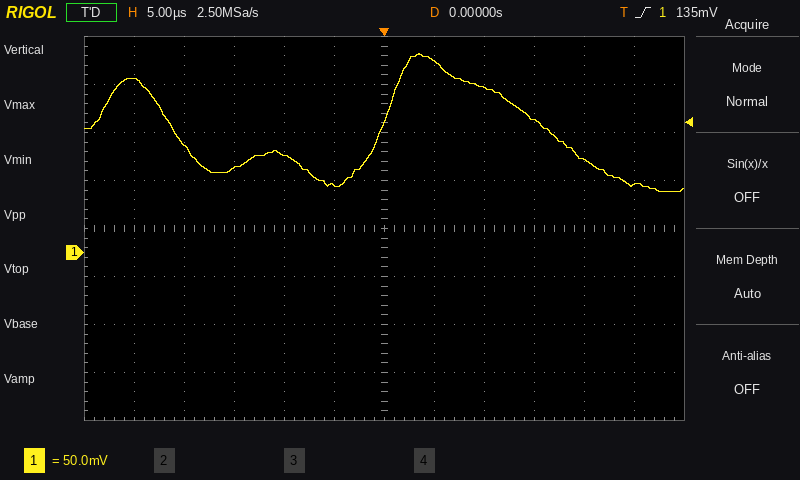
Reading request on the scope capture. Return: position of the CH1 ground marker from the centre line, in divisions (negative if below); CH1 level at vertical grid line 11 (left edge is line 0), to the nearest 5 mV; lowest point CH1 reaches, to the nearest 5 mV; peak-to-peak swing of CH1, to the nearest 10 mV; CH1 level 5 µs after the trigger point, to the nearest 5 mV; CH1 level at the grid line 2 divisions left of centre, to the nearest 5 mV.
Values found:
-0.5 div
70 mV
65 mV
140 mV
200 mV
100 mV
